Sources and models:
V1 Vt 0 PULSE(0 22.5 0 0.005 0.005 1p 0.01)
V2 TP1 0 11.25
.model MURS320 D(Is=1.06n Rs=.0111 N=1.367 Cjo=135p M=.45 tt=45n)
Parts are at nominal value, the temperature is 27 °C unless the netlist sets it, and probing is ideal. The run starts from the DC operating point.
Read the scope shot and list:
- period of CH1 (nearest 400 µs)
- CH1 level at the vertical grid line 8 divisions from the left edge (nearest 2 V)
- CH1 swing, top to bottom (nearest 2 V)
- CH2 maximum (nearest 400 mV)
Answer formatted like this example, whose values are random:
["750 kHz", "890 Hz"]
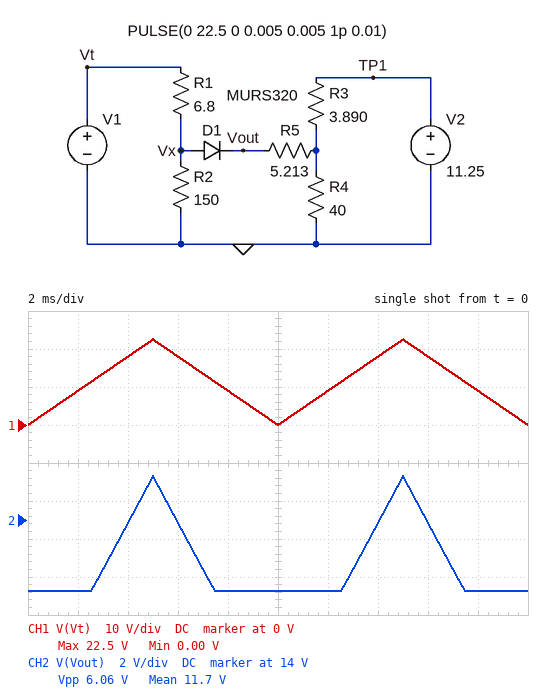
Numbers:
["10.0 ms", "18 V", "22 V", "16.4 V"]
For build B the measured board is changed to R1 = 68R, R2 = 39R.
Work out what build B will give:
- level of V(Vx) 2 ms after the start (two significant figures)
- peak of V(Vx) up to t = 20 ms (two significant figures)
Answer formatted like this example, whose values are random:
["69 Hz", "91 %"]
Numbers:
["3.3 V", "8.2 V"]
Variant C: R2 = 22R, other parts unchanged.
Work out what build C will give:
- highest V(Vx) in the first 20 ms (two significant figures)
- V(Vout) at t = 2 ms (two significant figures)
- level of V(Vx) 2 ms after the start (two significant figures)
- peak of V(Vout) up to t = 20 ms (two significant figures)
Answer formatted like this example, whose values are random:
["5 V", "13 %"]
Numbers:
["15 V", "10 V", "6.9 V", "14 V"]
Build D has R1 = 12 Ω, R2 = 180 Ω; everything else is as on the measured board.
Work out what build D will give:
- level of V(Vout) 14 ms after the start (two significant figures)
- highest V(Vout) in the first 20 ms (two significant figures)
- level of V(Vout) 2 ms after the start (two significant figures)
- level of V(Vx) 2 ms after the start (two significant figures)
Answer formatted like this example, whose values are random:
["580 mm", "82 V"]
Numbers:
["13 V", "15 V", "10 V", "8.4 V"]
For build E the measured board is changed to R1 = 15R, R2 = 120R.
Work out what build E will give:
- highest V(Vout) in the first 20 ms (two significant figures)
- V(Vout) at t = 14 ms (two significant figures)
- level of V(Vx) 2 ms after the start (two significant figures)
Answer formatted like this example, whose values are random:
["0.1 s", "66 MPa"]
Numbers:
["14 V", "12 V", "8.0 V"]
